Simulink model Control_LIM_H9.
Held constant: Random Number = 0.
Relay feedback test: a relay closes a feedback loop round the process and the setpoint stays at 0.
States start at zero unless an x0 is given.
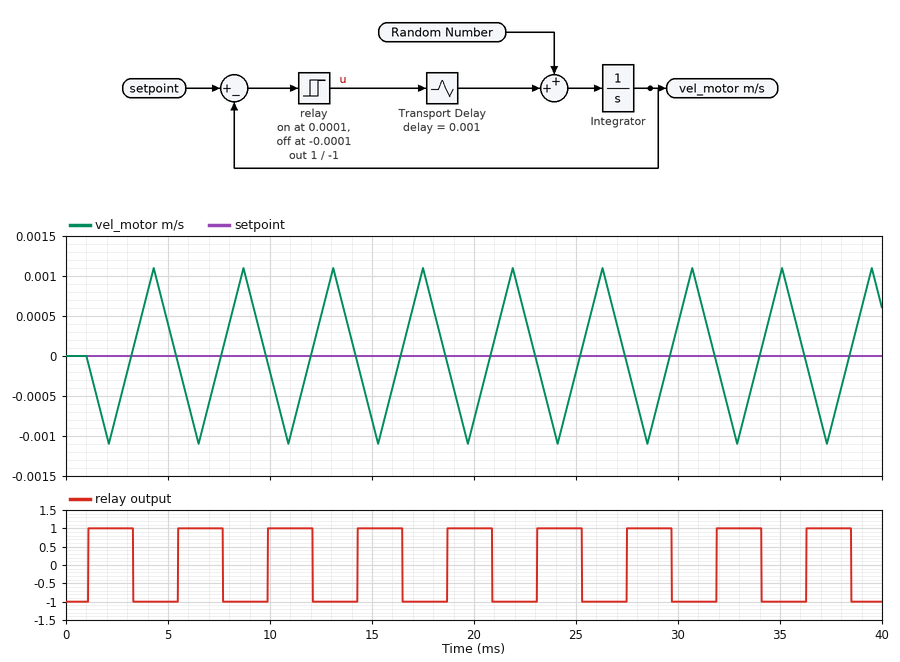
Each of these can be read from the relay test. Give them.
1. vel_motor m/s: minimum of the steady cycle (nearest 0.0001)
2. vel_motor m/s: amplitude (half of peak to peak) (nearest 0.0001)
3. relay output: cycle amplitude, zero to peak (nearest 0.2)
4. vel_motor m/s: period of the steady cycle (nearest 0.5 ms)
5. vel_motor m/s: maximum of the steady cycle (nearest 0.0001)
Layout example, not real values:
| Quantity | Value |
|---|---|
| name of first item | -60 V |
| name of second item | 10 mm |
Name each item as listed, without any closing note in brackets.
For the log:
| Quantity | Value |
|---|---|
| vel_motor m/s: minimum of the steady cycle | -0.0011 |
| vel_motor m/s: amplitude (half of peak to peak) | 0.0011 |
| relay output: cycle amplitude, zero to peak | 1.0 |
| vel_motor m/s: period of the steady cycle | 4.5 ms |
| vel_motor m/s: maximum of the steady cycle | 0.0011 |
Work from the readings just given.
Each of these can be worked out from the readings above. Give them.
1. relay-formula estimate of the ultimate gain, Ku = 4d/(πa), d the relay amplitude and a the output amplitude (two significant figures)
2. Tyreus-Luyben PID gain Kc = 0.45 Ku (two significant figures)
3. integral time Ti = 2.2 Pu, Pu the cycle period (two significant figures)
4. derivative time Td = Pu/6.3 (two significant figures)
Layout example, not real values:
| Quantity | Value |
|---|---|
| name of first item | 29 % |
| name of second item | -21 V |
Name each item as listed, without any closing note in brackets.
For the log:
| Quantity | Value |
|---|---|
| relay-formula estimate of the ultimate gain, Ku = 4d/(πa), d the relay amplitude and a the output amplitude | 1200 |
| Tyreus-Luyben PID gain Kc = 0.45 Ku | 540 |
| integral time Ti = 2.2 Pu, Pu the cycle period | 9.9 ms |
| derivative time Td = Pu/6.3 | 0.71 ms |
